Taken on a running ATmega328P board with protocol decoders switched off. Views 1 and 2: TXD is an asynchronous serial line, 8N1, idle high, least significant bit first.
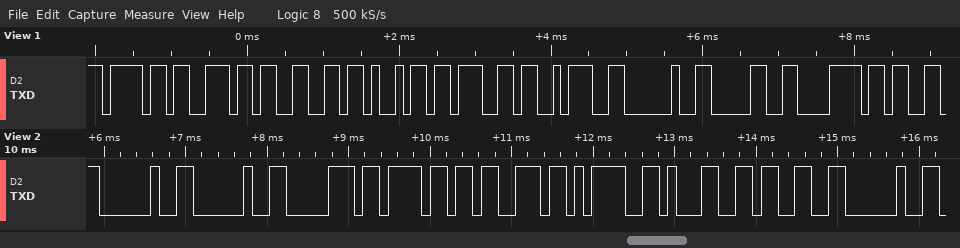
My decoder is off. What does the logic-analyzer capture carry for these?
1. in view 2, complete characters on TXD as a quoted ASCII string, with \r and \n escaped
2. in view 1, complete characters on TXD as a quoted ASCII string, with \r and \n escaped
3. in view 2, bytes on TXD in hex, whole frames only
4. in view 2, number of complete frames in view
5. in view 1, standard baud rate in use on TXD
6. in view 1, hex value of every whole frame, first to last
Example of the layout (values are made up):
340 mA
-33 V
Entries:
"  pos=13 "
"onfig: 0x"
20 20 70 6F 73 3D 31 33 20
9
9600 baud
0x6F 0x6E 0x66 0x69 0x67 0x3A 0x20 0x30 0x78
